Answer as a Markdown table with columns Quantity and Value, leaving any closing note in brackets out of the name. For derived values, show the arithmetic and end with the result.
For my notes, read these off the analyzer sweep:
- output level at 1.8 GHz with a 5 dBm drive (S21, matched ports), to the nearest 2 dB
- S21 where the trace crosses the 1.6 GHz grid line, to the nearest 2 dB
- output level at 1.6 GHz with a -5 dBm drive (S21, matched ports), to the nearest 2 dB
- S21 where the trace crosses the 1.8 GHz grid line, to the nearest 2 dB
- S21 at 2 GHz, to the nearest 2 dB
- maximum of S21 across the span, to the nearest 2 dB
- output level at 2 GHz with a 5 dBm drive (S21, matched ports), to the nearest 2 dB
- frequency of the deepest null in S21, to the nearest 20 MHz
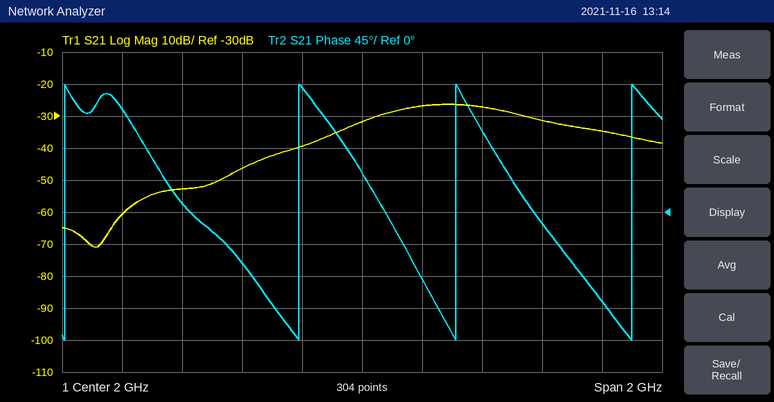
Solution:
| Quantity | Value |
|---|---|
| output level at 1.8 GHz with a 5 dBm drive (S21, matched ports), to the nearest 2 dB | 5 dBm + (-40 dB) = -34 dBm |
| S21 where the trace crosses the 1.6 GHz grid line, to the nearest 2 dB | -46 dB |
| output level at 1.6 GHz with a -5 dBm drive (S21, matched ports), to the nearest 2 dB | -5 dBm + (-46 dB) = -52 dBm |
| S21 where the trace crosses the 1.8 GHz grid line, to the nearest 2 dB | -40 dB |
| S21 at 2 GHz, to the nearest 2 dB | -32 dB |
| maximum of S21 across the span, to the nearest 2 dB | -26 dB |
| output level at 2 GHz with a 5 dBm drive (S21, matched ports), to the nearest 2 dB | 5 dBm + (-32 dB) = -26 dBm |
| frequency of the deepest null in S21, to the nearest 20 MHz | 1.12 GHz |
